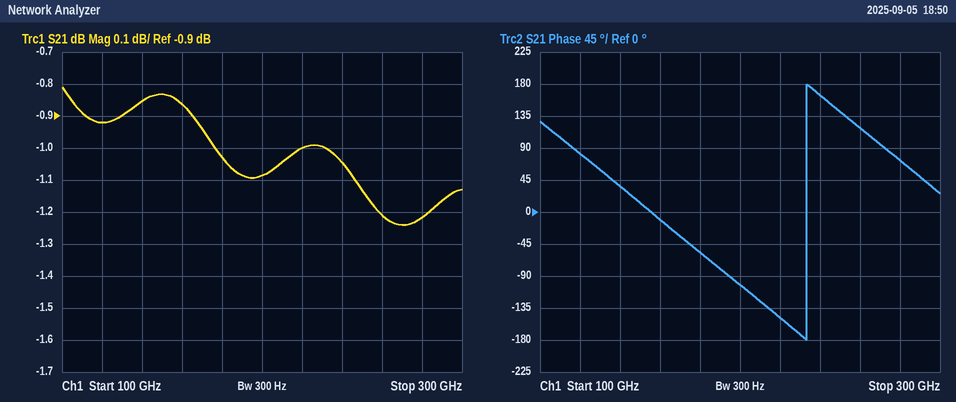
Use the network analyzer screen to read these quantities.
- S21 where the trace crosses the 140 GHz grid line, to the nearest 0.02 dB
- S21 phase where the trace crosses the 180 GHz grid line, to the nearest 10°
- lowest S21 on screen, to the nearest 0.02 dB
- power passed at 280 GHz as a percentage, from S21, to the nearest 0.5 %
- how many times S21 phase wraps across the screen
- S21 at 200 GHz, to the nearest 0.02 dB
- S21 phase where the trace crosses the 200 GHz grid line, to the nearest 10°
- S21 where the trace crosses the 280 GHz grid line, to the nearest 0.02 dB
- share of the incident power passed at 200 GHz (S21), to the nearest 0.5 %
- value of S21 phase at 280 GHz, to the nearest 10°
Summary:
-0.86 dB
-60°
-1.24 dB
75.5 %
1
-1.08 dB
-100°
-1.22 dB
78.0 %
70°
